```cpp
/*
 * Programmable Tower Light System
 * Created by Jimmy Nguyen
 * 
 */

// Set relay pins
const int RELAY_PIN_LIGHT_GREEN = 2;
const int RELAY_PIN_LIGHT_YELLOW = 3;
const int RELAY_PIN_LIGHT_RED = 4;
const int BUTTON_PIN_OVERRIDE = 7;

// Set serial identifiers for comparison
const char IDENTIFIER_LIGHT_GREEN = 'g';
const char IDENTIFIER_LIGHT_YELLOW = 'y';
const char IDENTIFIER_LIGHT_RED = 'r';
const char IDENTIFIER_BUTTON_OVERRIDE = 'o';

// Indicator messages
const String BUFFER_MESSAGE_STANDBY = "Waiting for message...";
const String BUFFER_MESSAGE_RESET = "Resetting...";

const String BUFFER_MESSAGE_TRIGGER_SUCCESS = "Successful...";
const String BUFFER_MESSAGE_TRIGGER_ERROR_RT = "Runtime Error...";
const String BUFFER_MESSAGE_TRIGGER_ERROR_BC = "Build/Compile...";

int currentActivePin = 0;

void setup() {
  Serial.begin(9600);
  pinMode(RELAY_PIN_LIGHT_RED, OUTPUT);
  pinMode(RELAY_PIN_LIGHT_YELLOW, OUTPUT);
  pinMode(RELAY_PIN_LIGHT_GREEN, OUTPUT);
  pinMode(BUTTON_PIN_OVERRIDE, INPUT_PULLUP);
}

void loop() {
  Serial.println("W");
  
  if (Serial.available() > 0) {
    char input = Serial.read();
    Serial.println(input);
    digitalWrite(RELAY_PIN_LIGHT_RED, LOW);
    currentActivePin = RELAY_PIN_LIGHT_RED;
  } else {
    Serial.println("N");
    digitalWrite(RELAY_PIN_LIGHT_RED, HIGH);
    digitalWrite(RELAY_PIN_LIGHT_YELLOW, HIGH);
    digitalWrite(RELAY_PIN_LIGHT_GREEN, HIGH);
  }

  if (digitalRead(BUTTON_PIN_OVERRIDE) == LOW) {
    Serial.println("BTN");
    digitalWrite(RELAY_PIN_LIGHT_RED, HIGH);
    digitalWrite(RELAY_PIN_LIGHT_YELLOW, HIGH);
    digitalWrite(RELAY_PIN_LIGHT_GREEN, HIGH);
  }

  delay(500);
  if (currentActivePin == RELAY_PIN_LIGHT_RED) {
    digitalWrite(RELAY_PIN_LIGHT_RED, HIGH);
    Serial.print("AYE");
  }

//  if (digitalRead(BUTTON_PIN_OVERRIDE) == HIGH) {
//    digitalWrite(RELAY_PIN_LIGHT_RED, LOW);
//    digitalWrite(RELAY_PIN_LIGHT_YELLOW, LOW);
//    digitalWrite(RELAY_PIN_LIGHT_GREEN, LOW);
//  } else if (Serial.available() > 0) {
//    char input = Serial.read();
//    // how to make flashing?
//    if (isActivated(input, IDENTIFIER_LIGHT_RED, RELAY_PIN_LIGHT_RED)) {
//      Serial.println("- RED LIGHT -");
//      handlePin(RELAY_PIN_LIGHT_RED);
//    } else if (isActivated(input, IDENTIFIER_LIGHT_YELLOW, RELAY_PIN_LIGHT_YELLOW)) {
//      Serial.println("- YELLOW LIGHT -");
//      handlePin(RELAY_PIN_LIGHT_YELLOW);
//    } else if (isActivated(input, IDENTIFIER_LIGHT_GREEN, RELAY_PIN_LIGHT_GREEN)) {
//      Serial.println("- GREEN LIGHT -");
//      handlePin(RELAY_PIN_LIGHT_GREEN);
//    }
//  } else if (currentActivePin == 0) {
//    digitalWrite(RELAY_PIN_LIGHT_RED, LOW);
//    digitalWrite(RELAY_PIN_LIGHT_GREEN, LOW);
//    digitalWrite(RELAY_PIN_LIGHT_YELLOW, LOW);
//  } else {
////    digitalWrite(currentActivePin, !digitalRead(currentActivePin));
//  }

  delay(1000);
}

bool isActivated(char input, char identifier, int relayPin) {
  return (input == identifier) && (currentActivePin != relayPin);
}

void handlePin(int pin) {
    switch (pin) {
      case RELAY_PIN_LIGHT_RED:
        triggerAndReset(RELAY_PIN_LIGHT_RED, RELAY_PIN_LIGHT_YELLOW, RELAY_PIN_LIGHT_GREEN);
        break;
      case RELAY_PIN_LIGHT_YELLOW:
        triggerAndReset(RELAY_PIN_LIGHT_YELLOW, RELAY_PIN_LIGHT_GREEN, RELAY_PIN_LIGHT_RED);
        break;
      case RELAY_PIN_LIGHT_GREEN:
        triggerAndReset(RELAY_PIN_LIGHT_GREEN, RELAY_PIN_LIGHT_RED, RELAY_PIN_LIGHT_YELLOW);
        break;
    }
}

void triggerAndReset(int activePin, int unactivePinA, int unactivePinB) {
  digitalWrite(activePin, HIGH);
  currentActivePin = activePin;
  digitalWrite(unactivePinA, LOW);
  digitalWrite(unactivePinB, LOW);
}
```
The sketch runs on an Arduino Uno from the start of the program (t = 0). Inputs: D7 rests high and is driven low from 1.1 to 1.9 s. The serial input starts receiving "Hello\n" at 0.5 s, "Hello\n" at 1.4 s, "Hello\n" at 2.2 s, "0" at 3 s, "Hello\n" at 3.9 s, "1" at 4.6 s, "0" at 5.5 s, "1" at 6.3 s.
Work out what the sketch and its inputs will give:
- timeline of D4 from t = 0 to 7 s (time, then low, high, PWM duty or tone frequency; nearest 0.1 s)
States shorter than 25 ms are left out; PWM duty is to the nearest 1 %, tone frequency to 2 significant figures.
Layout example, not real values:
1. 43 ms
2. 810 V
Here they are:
1. 0 s high; 3 s low; 3.5 s high; 4.5 s low; 5 s high; 6 s low; 6.5 s high
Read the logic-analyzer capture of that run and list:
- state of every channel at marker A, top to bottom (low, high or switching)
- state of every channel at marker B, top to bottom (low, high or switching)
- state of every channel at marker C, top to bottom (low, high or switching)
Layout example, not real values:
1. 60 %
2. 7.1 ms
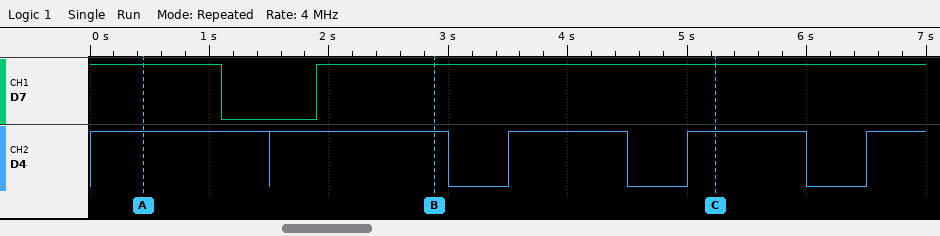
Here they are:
1. D7 high, D4 high
2. D7 high, D4 high
3. D7 high, D4 high
